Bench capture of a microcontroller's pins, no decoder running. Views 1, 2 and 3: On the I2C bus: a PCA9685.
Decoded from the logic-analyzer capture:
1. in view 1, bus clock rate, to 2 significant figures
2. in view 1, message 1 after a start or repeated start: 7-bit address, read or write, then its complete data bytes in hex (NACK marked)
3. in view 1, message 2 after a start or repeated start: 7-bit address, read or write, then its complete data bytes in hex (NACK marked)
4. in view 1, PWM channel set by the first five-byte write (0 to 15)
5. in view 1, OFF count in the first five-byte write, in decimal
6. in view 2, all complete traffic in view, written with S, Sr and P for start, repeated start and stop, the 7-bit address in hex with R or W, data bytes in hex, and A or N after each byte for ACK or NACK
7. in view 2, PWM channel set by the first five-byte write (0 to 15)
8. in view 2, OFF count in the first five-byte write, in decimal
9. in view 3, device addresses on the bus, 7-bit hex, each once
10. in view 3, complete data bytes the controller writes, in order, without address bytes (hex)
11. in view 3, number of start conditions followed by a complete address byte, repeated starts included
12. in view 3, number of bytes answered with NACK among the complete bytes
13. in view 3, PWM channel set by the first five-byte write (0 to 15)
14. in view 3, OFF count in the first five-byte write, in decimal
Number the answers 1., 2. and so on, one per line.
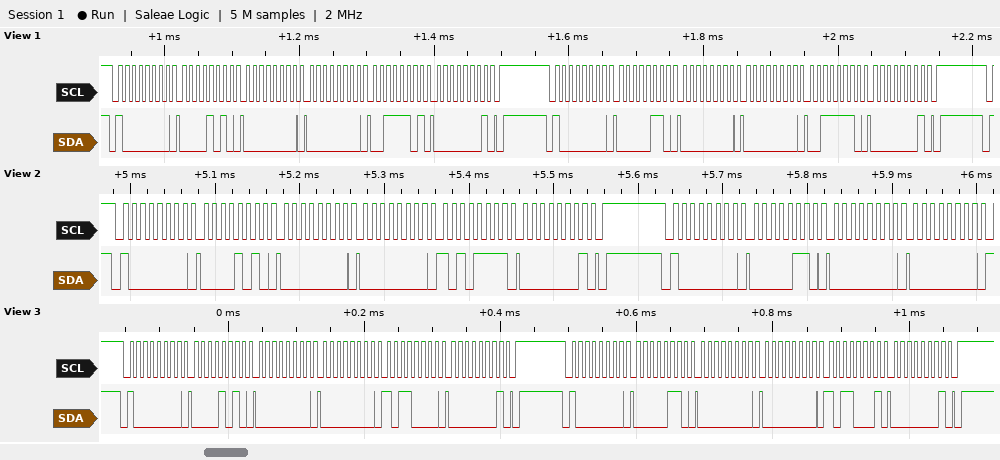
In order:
1. 100 kHz
2. 0x40 write: 0A 00 00 3D 01
3. 0x40 write: 06 00 00 3E 01
4. 1
5. 317
6. S 40W A 0A A 00 A 00 A AF A 01 A P S 40W A 06 A 00 A 00 A
7. 1
8. 431
9. 0x40
10. 0A 00 00 B0 01 06 00 00 B1 01
11. 2
12. 0
13. 1
14. 432
